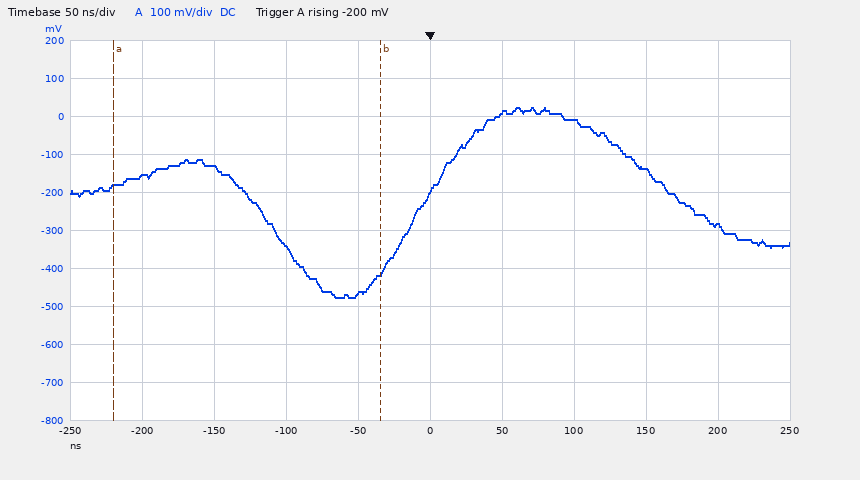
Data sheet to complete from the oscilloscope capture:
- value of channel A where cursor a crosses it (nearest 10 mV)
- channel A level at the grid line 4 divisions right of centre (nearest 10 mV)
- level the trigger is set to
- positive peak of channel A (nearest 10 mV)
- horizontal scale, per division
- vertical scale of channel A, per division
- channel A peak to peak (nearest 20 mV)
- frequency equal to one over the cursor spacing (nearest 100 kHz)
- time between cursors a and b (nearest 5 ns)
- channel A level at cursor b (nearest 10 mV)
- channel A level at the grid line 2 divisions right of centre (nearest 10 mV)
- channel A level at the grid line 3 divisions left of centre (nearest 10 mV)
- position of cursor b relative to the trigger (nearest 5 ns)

-180 mV
-290 mV
-200 mV
20 mV
50 ns
100 mV
500 mV
5.4 MHz
185 ns
-410 mV
-10 mV
-130 mV
-35 ns
